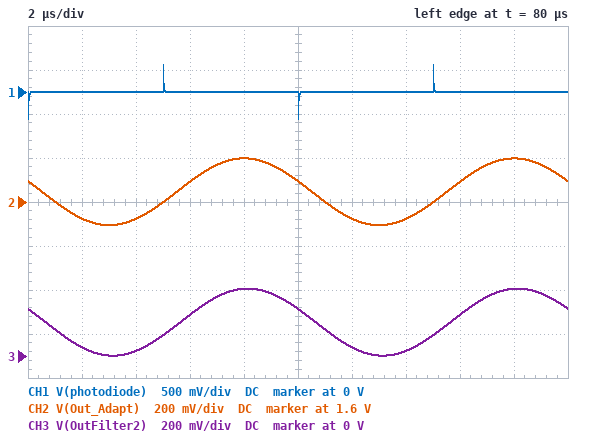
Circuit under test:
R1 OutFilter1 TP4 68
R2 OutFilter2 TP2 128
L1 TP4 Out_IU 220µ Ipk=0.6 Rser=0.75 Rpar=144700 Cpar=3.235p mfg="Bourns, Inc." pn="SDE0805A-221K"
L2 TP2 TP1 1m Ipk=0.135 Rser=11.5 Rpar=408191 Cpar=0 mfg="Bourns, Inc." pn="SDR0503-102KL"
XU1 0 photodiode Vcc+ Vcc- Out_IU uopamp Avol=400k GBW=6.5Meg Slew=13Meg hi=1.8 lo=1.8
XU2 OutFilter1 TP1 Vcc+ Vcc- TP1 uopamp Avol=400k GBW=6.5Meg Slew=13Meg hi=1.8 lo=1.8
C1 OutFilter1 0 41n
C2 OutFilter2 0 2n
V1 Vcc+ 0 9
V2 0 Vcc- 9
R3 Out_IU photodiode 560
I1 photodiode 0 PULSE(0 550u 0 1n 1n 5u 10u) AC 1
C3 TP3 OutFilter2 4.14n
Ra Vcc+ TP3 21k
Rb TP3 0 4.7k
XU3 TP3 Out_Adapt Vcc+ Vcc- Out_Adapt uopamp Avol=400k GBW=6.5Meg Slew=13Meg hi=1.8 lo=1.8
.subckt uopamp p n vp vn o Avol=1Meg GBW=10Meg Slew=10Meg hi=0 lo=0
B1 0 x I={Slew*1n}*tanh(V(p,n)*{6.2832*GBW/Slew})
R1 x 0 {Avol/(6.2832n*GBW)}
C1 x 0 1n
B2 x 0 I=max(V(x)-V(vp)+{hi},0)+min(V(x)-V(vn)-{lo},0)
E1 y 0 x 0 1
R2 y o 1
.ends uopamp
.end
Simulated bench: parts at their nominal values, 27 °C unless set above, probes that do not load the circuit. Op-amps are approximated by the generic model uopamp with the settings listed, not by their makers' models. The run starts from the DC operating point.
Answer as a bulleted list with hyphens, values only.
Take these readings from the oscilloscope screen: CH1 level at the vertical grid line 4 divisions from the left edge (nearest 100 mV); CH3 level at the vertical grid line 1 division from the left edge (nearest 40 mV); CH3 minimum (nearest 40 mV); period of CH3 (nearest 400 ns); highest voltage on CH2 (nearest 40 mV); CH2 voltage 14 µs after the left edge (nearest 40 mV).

- 0 V
- 40 mV
- 0 V
- 10.0 µs
- 1.80 V
- 1.52 V
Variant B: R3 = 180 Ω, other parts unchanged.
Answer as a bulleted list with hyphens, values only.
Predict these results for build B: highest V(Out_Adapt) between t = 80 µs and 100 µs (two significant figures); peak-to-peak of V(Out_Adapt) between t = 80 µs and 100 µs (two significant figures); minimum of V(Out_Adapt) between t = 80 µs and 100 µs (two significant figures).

- 1.7 V
- 98 mV
- 1.6 V
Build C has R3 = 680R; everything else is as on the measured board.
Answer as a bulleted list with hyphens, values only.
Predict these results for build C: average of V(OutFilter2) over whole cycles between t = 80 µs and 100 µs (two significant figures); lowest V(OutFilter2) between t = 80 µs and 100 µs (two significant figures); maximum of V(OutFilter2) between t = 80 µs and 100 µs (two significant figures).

- 190 mV
- 1.8 mV
- 370 mV
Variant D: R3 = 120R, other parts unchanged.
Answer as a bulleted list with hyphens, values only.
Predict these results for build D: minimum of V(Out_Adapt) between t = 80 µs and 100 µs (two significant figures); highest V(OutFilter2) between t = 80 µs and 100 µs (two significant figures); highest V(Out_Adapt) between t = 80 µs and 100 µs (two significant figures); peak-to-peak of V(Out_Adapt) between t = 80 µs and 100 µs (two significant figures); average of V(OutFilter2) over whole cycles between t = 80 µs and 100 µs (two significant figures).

- 1.6 V
- 66 mV
- 1.7 V
- 65 mV
- 33 mV
